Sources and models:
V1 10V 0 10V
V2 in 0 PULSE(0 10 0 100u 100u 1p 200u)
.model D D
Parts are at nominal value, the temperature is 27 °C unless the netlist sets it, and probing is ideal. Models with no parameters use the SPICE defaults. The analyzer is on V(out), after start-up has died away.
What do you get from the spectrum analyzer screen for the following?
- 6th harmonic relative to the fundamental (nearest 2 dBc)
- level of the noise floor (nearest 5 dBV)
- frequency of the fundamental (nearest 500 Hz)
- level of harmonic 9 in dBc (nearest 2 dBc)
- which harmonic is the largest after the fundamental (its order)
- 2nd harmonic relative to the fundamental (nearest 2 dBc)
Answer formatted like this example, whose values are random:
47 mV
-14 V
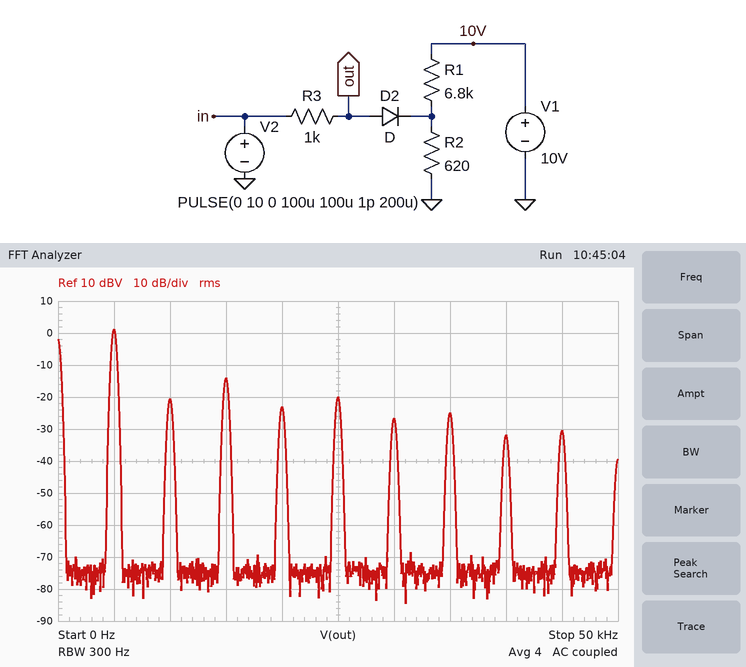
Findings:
-28 dBc
-75 dBV
5.0 kHz
-32 dBc
3
-22 dBc
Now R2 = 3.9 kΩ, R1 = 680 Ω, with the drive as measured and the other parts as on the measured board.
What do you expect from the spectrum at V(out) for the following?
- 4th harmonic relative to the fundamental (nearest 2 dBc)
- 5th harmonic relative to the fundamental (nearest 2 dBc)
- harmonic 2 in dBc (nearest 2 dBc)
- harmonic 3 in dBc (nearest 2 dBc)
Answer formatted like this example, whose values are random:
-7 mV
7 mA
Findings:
-40 dBc
-30 dBc
-38 dBc
-20 dBc
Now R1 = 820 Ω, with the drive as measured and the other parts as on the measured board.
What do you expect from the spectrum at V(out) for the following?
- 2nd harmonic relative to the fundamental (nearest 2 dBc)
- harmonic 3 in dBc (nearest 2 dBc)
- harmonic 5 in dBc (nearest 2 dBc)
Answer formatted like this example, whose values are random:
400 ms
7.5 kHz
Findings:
-10 dBc
-18 dBc
-28 dBc
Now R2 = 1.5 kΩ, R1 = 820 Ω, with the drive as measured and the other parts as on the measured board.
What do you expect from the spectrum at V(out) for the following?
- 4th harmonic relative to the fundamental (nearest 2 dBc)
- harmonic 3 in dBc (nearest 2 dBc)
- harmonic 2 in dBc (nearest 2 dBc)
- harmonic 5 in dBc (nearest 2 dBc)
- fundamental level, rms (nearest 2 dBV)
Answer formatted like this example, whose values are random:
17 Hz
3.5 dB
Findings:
-28 dBc
-26 dBc
-18 dBc
-30 dBc
8 dBV
